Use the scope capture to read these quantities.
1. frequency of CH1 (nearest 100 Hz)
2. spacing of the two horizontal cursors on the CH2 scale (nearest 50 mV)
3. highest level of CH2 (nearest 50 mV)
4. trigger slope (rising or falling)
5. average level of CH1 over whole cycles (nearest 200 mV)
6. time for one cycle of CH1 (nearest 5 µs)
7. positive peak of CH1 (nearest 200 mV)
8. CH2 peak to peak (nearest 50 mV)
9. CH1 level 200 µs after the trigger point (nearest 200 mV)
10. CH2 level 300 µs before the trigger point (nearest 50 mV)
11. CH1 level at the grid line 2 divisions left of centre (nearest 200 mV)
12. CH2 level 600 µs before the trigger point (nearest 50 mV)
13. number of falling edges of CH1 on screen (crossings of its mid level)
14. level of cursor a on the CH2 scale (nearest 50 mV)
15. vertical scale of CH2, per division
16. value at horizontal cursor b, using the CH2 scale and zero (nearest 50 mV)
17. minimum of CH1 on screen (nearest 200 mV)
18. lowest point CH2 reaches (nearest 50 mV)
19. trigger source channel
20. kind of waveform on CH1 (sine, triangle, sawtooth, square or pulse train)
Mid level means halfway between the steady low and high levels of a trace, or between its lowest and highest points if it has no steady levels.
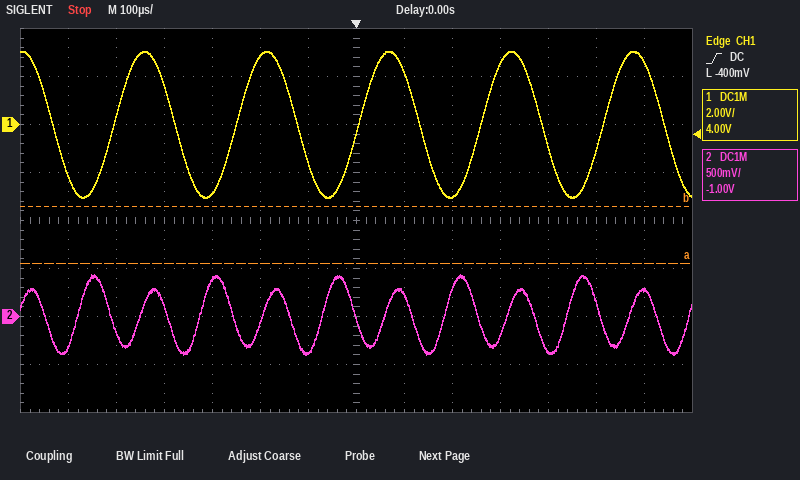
3.9 kHz
600 mV
450 mV
rising
0.0 V
255 µs
3.0 V
850 mV
-3.0 V
400 mV
2.8 V
-300 mV
6
550 mV
500 mV
1.15 V
-3.0 V
-400 mV
CH1
sine
